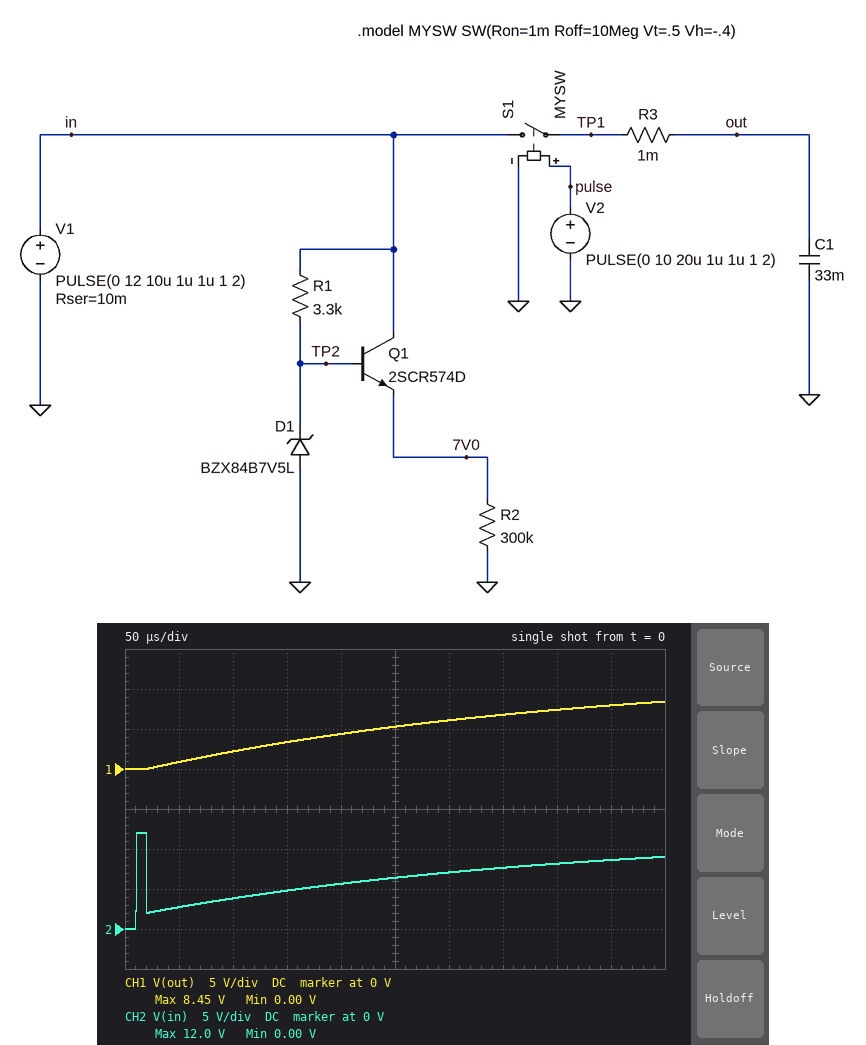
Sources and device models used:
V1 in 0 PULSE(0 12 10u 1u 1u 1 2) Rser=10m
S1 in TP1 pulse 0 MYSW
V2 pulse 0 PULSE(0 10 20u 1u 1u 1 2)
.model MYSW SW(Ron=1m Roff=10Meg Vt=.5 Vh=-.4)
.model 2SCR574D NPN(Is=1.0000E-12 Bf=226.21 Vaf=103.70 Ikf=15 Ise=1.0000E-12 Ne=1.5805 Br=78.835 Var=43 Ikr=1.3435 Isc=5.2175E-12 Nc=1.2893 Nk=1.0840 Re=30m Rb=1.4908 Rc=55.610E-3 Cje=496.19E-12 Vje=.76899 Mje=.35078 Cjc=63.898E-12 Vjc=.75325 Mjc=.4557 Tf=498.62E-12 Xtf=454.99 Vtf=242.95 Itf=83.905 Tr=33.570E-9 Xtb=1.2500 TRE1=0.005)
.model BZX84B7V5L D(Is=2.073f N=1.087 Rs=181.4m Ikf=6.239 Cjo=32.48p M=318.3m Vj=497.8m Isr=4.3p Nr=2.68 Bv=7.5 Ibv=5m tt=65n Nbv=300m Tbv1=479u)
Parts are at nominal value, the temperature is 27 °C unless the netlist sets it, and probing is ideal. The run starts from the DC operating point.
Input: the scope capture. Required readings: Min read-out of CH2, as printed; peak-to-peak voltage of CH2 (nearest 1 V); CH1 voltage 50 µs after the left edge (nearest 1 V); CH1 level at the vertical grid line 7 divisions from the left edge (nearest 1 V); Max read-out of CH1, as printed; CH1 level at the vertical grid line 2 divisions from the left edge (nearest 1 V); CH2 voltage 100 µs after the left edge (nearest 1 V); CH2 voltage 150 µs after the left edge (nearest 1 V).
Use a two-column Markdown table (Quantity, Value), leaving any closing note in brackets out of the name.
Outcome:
| Quantity | Value |
|---|---|
| Min read-out of CH2, as printed | 0.00 V |
| peak-to-peak voltage of CH2 | 12 V |
| CH1 voltage 50 µs after the left edge | 1 V |
| CH1 level at the vertical grid line 7 divisions from the left edge | 7 V |
| Max read-out of CH1, as printed | 8.45 V |
| CH1 level at the vertical grid line 2 divisions from the left edge | 2 V |
| CH2 voltage 100 µs after the left edge | 4 V |
| CH2 voltage 150 µs after the left edge | 5 V |
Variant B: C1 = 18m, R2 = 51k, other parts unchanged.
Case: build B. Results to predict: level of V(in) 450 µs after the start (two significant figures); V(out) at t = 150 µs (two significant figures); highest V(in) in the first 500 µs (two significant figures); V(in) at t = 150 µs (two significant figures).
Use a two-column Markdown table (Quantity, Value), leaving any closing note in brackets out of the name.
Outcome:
| Quantity | Value |
|---|---|
| level of V(in) 450 µs after the start | 11 V |
| V(out) at t = 150 µs | 5.4 V |
| highest V(in) in the first 500 µs | 12 V |
| V(in) at t = 150 µs | 6.5 V |
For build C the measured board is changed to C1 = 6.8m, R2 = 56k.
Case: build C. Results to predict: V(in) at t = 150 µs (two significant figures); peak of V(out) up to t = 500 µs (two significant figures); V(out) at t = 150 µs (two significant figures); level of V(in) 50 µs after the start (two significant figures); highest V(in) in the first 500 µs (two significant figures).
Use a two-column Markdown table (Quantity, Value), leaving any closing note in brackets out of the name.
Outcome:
| Quantity | Value |
|---|---|
| V(in) at t = 150 µs | 10 V |
| peak of V(out) up to t = 500 µs | 12 V |
| V(out) at t = 150 µs | 9.6 V |
| level of V(in) 50 µs after the start | 5.1 V |
| highest V(in) in the first 500 µs | 12 V |
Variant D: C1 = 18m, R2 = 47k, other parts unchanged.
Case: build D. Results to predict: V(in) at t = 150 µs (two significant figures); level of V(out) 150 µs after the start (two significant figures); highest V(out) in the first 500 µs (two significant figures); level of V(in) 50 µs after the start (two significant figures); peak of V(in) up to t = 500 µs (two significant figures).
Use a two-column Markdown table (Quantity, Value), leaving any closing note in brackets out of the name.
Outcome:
| Quantity | Value |
|---|---|
| V(in) at t = 150 µs | 6.5 V |
| level of V(out) 150 µs after the start | 5.4 V |
| highest V(out) in the first 500 µs | 11 V |
| level of V(in) 50 µs after the start | 3.3 V |
| peak of V(in) up to t = 500 µs | 12 V |
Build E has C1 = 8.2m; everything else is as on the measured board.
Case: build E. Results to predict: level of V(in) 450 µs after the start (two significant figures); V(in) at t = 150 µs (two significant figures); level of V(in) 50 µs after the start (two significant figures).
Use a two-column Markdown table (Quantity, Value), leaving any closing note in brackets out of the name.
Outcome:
| Quantity | Value |
|---|---|
| level of V(in) 450 µs after the start | 12 V |
| V(in) at t = 150 µs | 9.3 V |
| level of V(in) 50 µs after the start | 4.6 V |
